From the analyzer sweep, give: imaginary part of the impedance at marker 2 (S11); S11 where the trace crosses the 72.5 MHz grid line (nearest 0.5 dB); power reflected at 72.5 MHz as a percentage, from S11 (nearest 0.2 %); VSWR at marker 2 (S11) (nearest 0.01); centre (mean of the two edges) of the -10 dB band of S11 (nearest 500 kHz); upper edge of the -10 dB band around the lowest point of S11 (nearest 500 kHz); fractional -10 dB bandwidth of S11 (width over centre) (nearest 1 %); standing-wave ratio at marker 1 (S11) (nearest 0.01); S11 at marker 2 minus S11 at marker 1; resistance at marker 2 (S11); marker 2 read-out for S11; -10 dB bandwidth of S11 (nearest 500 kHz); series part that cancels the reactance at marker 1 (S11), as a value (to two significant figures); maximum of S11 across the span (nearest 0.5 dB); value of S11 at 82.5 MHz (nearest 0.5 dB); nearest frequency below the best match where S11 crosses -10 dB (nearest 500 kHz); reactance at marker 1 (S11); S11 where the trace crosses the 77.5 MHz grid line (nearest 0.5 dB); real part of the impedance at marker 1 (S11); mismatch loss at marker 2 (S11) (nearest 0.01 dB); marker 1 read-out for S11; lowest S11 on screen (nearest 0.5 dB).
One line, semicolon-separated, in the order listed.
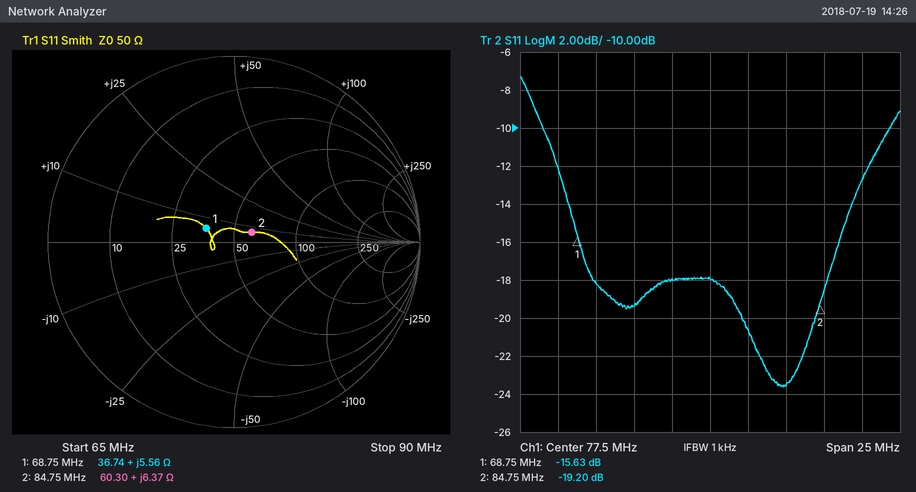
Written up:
+6.37 Ω; -19.5 dB; 1.2 %; 1.25; 78.0 MHz; 89.5 MHz; 29 %; 1.40; -3.57 dB; 60.30 Ω; -19.20 dB; 23.0 MHz; 420 pF; -7.5 dB; -23.5 dB; 66.5 MHz; +5.56 Ω; -18.0 dB; 36.74 Ω; 0.05 dB; -15.63 dB; -23.5 dB
